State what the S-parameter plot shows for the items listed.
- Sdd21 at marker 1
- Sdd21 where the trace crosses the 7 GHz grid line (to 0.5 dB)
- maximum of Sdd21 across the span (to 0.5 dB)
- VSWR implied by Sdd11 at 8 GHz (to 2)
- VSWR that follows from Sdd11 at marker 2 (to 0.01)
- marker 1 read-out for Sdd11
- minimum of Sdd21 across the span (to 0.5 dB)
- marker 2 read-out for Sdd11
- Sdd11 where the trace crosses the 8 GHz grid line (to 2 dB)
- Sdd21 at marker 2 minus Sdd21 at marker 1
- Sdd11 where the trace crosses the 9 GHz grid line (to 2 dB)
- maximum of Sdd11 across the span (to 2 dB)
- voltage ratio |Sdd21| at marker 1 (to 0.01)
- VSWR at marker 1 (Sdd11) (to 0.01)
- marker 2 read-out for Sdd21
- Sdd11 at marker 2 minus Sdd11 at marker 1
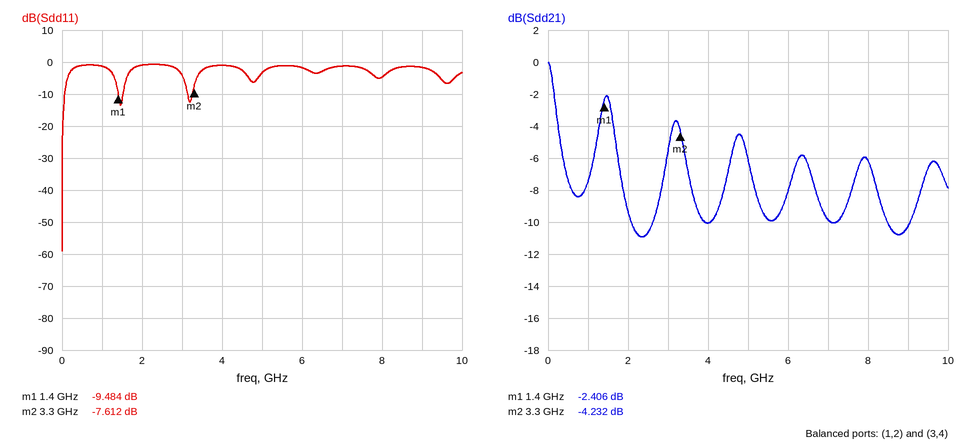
-2.406 dB
-10.0 dB
0.0 dB
4
2.43
-9.484 dB
-11.0 dB
-7.612 dB
-4 dB
-1.826 dB
-2 dB
0 dB
0.76
2.01
-4.232 dB
1.872 dB
